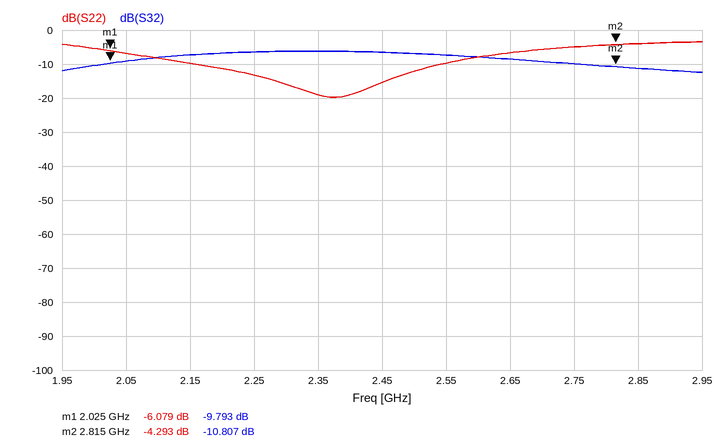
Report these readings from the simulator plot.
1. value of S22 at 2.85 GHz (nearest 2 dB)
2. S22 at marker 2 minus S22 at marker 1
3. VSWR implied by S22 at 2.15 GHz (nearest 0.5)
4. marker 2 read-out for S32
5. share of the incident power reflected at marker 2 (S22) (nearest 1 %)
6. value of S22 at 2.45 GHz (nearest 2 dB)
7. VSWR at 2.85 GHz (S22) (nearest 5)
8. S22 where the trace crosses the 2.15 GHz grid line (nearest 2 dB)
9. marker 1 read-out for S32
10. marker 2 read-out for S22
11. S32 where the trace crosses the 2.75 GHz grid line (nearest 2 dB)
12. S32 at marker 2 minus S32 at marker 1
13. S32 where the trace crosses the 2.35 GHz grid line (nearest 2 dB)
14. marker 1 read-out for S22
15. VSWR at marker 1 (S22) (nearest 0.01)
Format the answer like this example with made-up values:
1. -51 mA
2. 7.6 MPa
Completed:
1. -4 dB
2. 1.786 dB
3. 2.0
4. -10.807 dB
5. 37 %
6. -16 dB
7. 5
8. -10 dB
9. -9.793 dB
10. -4.293 dB
11. -10 dB
12. -1.014 dB
13. -6 dB
14. -6.079 dB
15. 2.97
